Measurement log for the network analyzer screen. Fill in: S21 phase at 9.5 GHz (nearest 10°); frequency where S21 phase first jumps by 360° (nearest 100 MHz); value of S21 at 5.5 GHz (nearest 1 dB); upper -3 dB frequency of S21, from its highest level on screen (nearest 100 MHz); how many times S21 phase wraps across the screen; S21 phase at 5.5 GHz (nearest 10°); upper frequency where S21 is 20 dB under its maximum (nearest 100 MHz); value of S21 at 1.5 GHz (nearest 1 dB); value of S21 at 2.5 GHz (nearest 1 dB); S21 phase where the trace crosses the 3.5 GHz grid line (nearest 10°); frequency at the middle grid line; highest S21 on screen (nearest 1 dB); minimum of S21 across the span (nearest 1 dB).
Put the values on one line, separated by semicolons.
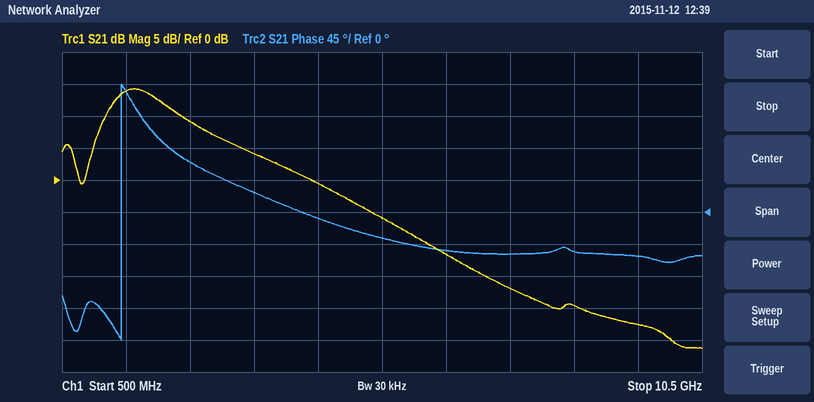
-60°; 1.4 GHz; -6 dB; 2.2 GHz; 1; -40°; 5.5 GHz; 14 dB; 9 dB; 30°; 5.5 GHz; 14 dB; -26 dB
